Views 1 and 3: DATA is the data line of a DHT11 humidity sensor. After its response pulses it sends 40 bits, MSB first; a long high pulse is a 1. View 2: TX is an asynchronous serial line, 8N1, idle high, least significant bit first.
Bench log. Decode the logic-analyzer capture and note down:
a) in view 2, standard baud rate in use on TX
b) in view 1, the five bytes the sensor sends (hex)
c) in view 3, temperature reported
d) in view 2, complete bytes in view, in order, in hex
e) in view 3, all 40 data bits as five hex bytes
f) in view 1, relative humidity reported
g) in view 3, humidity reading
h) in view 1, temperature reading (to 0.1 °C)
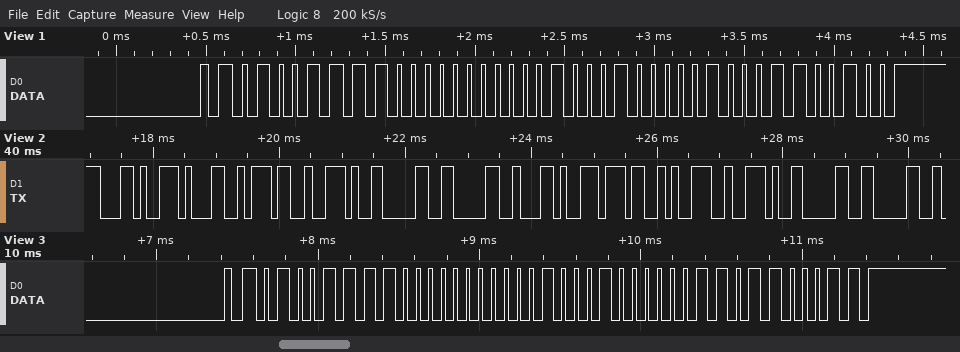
9600 baud
4F 00 11 04 64
17.3 °C
2C 31 37 2E 30 30 2C 37 39 2E 30 30
4F 00 11 03 63
79 %
79 %
17.4 °C
